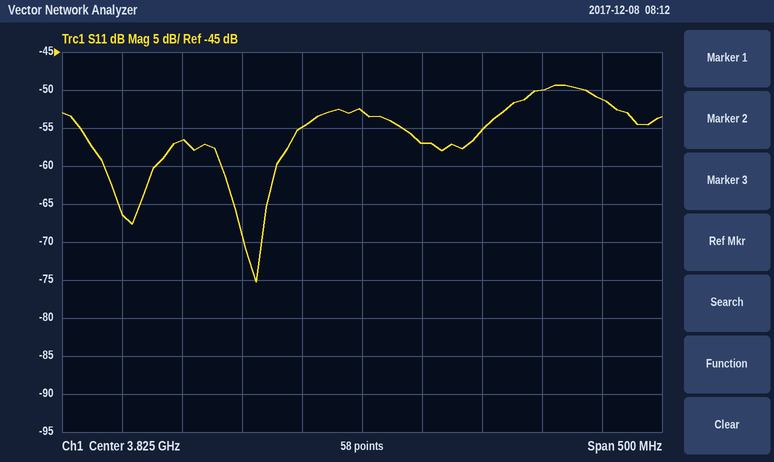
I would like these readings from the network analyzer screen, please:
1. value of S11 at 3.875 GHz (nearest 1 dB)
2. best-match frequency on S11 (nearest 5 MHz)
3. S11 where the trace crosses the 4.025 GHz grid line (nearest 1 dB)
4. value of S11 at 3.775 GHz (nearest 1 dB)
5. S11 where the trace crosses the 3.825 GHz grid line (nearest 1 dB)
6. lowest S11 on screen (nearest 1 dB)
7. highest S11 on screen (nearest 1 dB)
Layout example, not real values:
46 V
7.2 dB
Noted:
-57 dB
3.735 GHz
-51 dB
-55 dB
-53 dB
-75 dB
-49 dB
